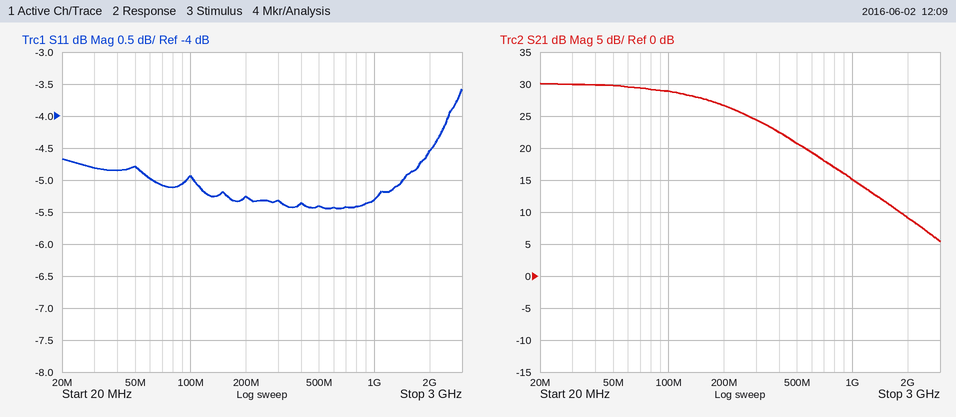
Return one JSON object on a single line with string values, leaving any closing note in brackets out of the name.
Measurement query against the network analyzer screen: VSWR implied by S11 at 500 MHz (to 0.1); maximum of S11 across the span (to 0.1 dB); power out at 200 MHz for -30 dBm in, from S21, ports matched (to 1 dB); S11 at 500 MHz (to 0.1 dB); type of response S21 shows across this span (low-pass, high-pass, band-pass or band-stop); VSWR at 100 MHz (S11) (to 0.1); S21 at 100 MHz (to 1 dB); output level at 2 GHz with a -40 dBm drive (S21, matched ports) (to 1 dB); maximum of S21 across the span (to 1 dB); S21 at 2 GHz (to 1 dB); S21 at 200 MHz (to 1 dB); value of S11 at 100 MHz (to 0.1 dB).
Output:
{"VSWR implied by S11 at 500 MHz": "3.3", "maximum of S11 across the span": "-3.6 dB", "power out at 200 MHz for -30 dBm in, from S21, ports matched": "-3 dBm", "S11 at 500 MHz": "-5.4 dB", "type of response S21 shows across this span": "low-pass", "VSWR at 100 MHz (S11)": "3.6", "S21 at 100 MHz": "29 dB", "output level at 2 GHz with a -40 dBm drive (S21, matched ports)": "-31 dBm", "maximum of S21 across the span": "30 dB", "S21 at 2 GHz": "9 dB", "S21 at 200 MHz": "27 dB", "value of S11 at 100 MHz": "-4.9 dB"}
